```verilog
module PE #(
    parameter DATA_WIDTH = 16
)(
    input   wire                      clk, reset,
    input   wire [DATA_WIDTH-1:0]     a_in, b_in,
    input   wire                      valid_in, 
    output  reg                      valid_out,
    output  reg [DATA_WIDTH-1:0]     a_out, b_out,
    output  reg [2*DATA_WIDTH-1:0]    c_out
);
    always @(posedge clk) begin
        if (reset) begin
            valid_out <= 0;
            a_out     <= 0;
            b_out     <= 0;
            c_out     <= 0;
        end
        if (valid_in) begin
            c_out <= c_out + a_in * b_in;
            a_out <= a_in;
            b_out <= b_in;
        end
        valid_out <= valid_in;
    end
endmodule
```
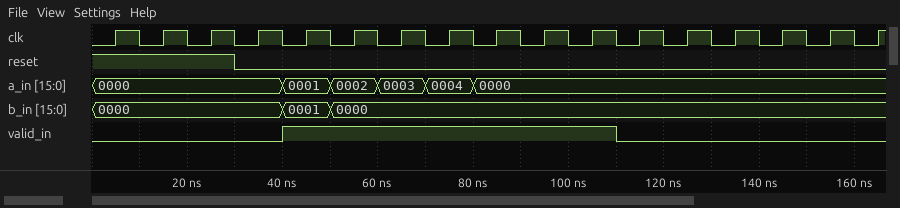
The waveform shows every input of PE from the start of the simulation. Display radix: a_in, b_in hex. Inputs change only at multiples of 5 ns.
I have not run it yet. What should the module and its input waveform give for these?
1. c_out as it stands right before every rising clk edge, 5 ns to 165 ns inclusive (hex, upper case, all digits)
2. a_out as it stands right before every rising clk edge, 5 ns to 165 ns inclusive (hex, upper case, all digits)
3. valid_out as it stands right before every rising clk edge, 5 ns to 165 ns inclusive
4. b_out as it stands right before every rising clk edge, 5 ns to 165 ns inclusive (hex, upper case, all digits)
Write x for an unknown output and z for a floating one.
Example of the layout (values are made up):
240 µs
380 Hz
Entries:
x, 00000000, 00000000, 00000000, 00000000, 00000001, 00000001, 00000001, 00000001, 00000001, 00000001, 00000001, 00000001, 00000001, 00000001, 00000001, 00000001
x, 0000, 0000, 0000, 0000, 0001, 0002, 0003, 0004, 0000, 0000, 0000, 0000, 0000, 0000, 0000, 0000
x 0 0 0 0 1 1 1 1 1 1 1 0 0 0 0 0
x, 0000, 0000, 0000, 0000, 0001, 0000, 0000, 0000, 0000, 0000, 0000, 0000, 0000, 0000, 0000, 0000
